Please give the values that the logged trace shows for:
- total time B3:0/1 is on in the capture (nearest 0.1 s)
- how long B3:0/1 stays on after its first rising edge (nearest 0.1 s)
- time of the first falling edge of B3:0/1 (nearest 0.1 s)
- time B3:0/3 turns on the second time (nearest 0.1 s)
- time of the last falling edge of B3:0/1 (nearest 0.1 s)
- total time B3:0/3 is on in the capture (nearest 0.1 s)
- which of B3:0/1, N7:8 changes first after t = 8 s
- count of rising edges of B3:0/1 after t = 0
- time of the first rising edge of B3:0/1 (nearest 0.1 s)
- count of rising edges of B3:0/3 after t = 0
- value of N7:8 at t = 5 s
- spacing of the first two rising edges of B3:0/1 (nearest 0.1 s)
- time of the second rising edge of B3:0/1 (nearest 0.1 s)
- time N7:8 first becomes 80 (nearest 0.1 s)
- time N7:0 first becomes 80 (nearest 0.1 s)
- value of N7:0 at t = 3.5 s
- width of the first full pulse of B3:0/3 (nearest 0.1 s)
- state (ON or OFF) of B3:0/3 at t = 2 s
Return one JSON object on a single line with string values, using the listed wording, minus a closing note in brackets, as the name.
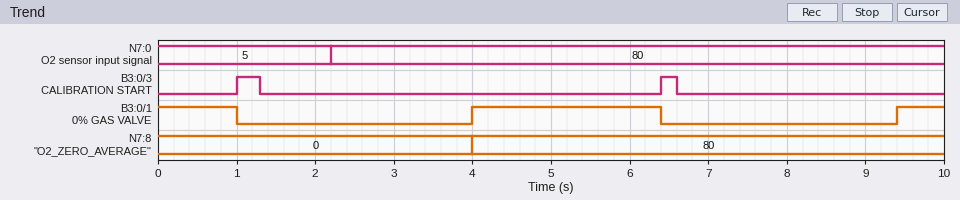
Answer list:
{"total time B3:0/1 is on in the capture": "4.0 s", "how long B3:0/1 stays on after its first rising edge": "2.4 s", "time of the first falling edge of B3:0/1": "1.0 s", "time B3:0/3 turns on the second time": "6.4 s", "time of the last falling edge of B3:0/1": "6.4 s", "total time B3:0/3 is on in the capture": "0.5 s", "which of B3:0/1, N7:8 changes first after t = 8 s": "B3:0/1", "count of rising edges of B3:0/1 after t = 0": "2", "time of the first rising edge of B3:0/1": "4.0 s", "count of rising edges of B3:0/3 after t = 0": "2", "value of N7:8 at t = 5 s": "80", "spacing of the first two rising edges of B3:0/1": "5.4 s", "time of the second rising edge of B3:0/1": "9.4 s", "time N7:8 first becomes 80": "4.0 s", "time N7:0 first becomes 80": "2.2 s", "value of N7:0 at t = 3.5 s": "80", "width of the first full pulse of B3:0/3": "0.3 s", "state (ON or OFF) of B3:0/3 at t = 2 s": "OFF"}
